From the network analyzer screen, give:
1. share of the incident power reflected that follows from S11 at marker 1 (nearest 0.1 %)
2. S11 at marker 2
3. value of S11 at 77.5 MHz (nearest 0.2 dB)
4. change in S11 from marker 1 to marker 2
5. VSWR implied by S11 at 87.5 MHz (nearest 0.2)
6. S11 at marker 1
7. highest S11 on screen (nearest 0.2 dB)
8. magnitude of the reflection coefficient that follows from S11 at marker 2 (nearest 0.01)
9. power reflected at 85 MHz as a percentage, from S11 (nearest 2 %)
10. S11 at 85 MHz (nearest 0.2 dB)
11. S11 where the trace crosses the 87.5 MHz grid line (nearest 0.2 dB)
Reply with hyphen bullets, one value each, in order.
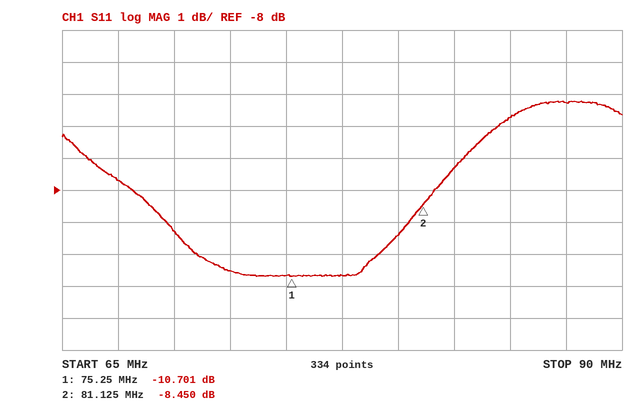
- 8.5 %
- -8.450 dB
- -10.6 dB
- 2.251 dB
- 3.4
- -10.701 dB
- -5.2 dB
- 0.38
- 26 %
- -5.8 dB
- -5.2 dB
